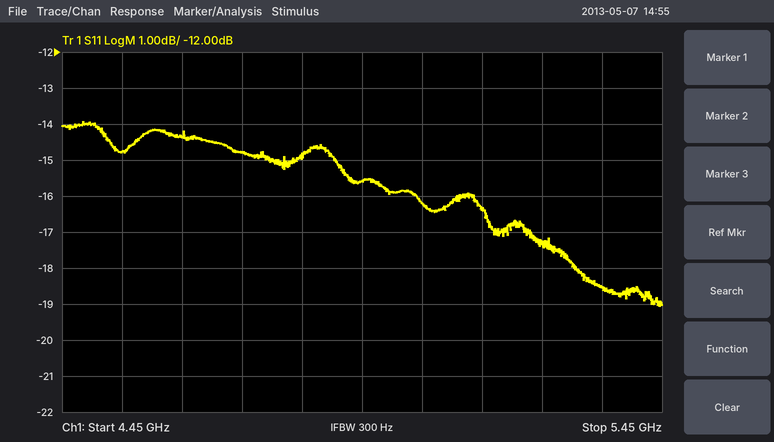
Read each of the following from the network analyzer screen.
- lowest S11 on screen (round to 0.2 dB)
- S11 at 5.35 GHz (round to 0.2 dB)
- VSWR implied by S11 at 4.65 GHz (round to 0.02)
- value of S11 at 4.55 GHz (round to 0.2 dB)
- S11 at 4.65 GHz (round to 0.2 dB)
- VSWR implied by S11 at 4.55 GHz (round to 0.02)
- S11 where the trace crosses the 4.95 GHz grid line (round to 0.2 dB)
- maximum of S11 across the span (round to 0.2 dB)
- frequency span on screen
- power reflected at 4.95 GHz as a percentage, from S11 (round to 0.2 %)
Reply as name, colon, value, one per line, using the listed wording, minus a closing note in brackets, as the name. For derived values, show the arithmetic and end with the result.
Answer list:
lowest S11 on screen: -19.0 dB
S11 at 5.35 GHz: -18.6 dB
VSWR implied by S11 at 4.65 GHz: |Γ| = 10^(-14.4/20) = 0.1905; VSWR = (1 + 0.1905)/(1 − 0.1905) ≈ 1.47, so 1.48 to the nearest 0.02
value of S11 at 4.55 GHz: -14.8 dB
S11 at 4.65 GHz: -14.4 dB
VSWR implied by S11 at 4.55 GHz: |Γ| = 10^(-14.8/20) = 0.1820; VSWR = (1 + 0.1820)/(1 − 0.1820) ≈ 1.44
S11 where the trace crosses the 4.95 GHz grid line: -15.6 dB
maximum of S11 across the span: -14.0 dB
frequency span on screen: 1 GHz
power reflected at 4.95 GHz as a percentage, from S11: 10^(-15.6/10) ≈ 2.8 %
